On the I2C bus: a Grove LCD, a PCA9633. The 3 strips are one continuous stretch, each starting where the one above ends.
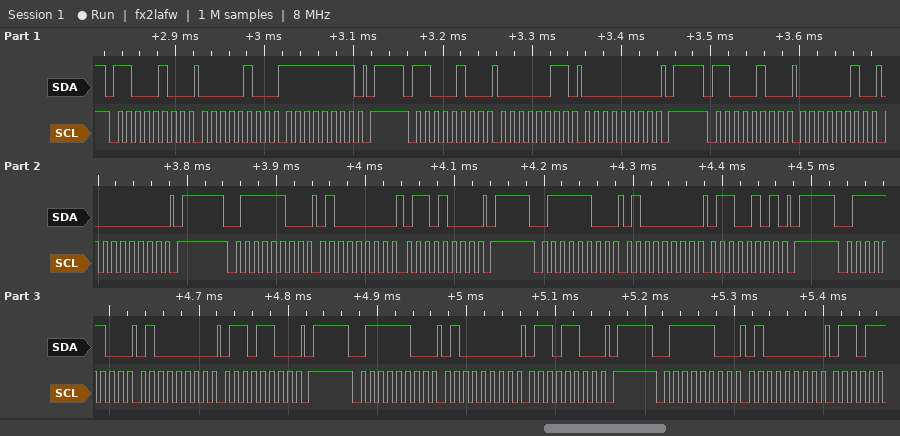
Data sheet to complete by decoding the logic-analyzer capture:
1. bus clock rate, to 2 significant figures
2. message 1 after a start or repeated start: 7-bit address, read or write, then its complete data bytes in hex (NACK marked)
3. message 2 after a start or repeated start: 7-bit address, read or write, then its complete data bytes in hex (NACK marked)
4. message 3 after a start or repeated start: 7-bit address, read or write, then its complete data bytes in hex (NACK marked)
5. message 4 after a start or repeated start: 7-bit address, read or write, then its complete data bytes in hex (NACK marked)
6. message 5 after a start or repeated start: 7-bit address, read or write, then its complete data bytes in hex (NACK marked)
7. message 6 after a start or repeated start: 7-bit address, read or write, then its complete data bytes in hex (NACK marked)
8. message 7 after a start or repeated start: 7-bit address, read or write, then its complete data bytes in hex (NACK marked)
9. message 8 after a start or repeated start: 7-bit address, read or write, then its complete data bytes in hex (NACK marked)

100 kHz
0x62 write: 04 FF
0x62 write: 03 00
0x62 write: 02 00
0x3E write: 40 68
0x3E write: 40 65
0x3E write: 40 6C
0x3E write: 40 6C
0x3E write: 40
